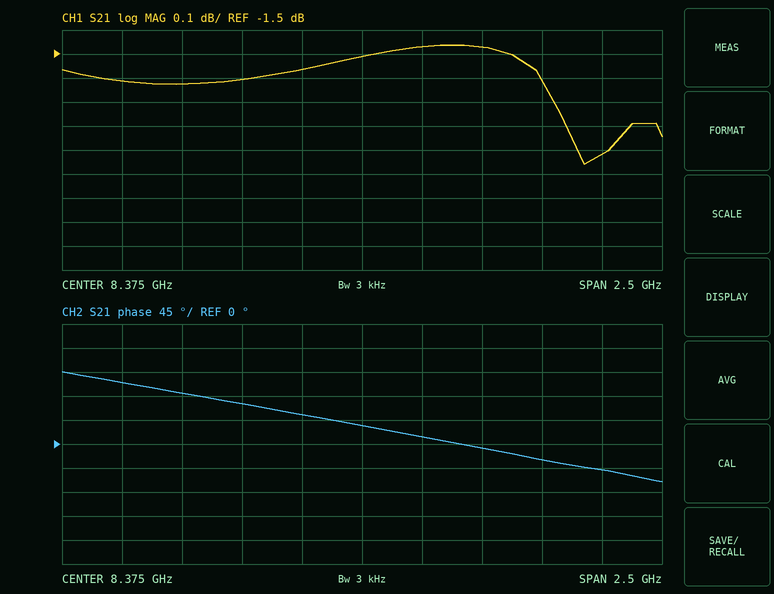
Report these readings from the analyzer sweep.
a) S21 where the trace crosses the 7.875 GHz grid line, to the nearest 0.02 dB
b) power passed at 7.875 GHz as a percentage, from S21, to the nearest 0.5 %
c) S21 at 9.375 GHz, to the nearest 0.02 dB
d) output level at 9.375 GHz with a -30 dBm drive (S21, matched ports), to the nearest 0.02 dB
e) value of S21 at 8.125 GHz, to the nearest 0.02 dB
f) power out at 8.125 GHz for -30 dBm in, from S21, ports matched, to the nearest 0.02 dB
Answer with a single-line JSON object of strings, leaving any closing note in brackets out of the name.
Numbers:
{"S21 where the trace crosses the 7.875 GHz grid line, to the nearest 0.02 dB": "-1.60 dB", "power passed at 7.875 GHz as a percentage, from S21, to the nearest 0.5 %": "69.0 %", "S21 at 9.375 GHz, to the nearest 0.02 dB": "-1.92 dB", "output level at 9.375 GHz with a -30 dBm drive (S21, matched ports), to the nearest 0.02 dB": "-31.92 dBm", "value of S21 at 8.125 GHz, to the nearest 0.02 dB": "-1.56 dB", "power out at 8.125 GHz for -30 dBm in, from S21, ports matched, to the nearest 0.02 dB": "-31.56 dBm"}
